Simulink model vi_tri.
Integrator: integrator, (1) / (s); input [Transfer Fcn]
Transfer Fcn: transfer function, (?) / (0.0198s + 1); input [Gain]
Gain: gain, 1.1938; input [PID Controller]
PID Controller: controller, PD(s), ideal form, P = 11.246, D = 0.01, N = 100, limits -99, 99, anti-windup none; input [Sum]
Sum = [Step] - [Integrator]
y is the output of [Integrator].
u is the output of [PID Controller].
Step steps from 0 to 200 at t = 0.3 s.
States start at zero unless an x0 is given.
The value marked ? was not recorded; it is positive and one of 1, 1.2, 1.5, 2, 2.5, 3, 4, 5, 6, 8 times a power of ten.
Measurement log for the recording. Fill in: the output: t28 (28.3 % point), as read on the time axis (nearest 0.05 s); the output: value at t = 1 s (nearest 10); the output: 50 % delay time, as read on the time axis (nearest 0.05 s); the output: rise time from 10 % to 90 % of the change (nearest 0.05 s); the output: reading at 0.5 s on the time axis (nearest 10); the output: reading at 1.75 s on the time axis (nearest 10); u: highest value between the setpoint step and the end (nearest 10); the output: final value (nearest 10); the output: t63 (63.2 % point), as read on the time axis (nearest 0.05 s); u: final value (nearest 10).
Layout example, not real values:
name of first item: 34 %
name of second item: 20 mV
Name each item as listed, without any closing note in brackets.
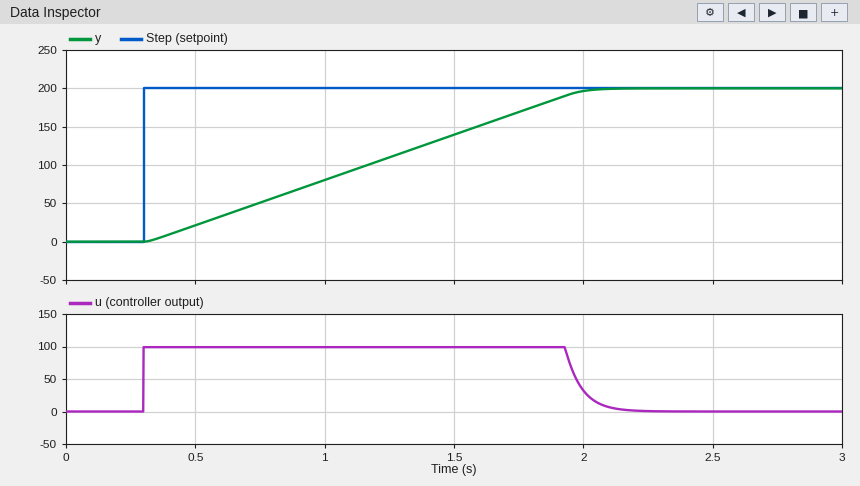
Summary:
the output: t28 (28.3 % point), as read on the time axis: 0.80 s
the output: value at t = 1 s: 80
the output: 50 % delay time, as read on the time axis: 1.15 s
the output: rise time from 10 % to 90 % of the change: 1.35 s
the output: reading at 0.5 s on the time axis: 20
the output: reading at 1.75 s on the time axis: 170
u: highest value between the setpoint step and the end: 100
the output: final value: 200
the output: t63 (63.2 % point), as read on the time axis: 1.40 s
u: final value: 0
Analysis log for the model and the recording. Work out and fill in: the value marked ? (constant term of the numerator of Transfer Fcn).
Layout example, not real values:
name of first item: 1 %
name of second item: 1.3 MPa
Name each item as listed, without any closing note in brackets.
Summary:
the value marked ?: 1
